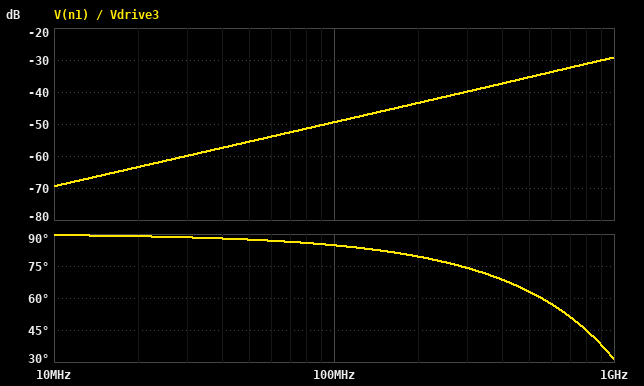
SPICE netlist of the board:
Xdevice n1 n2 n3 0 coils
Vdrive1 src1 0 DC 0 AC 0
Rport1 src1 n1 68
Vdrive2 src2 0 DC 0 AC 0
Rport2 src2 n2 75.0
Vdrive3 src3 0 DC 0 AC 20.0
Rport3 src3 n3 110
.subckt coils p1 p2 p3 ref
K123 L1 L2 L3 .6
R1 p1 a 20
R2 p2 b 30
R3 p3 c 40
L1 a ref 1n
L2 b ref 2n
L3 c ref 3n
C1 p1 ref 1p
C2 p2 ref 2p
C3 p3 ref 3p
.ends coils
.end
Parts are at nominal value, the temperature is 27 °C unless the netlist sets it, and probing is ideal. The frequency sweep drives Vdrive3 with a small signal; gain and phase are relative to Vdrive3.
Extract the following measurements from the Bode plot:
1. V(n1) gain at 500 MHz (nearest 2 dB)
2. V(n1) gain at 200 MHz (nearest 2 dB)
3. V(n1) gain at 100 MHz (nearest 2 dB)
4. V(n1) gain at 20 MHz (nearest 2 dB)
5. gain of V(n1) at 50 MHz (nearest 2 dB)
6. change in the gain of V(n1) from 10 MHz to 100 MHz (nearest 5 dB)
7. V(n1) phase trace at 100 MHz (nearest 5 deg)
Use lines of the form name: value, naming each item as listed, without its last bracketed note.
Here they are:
V(n1) gain at 500 MHz: -36 dB
V(n1) gain at 200 MHz: -44 dB
V(n1) gain at 100 MHz: -50 dB
V(n1) gain at 20 MHz: -64 dB
gain of V(n1) at 50 MHz: -56 dB
change in the gain of V(n1) from 10 MHz to 100 MHz: 20 dB
V(n1) phase trace at 100 MHz: 85 deg
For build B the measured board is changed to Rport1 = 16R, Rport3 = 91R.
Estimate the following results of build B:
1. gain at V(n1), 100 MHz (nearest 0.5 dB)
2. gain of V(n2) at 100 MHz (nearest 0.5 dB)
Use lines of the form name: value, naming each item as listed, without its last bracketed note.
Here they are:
gain at V(n1), 100 MHz: -53.0 dB
gain of V(n2) at 100 MHz: -46.0 dB
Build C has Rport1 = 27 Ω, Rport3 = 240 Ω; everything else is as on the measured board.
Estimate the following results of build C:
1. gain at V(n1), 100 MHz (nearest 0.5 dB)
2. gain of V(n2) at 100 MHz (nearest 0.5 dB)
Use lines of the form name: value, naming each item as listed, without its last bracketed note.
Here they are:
gain at V(n1), 100 MHz: -57.5 dB
gain of V(n2) at 100 MHz: -52.5 dB
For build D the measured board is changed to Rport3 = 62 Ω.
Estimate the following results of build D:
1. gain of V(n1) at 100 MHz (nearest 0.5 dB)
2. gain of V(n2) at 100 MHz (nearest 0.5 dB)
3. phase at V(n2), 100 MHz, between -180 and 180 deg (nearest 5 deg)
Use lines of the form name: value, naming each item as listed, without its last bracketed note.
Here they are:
gain of V(n1) at 100 MHz: -46.0 dB
gain of V(n2) at 100 MHz: -44.0 dB
phase at V(n2), 100 MHz, between -180 and 180 deg: 85 deg
